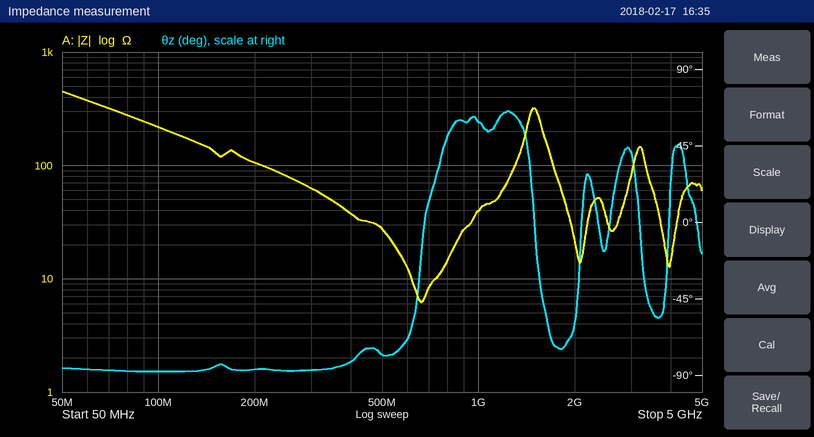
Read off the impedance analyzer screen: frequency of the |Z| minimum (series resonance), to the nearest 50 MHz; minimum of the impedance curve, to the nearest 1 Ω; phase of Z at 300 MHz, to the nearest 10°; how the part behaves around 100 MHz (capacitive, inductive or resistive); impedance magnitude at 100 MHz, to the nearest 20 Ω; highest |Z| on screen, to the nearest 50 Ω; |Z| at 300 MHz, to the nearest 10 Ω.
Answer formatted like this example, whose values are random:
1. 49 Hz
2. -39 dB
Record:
1. 650 MHz
2. 6 Ω
3. -90°
4. capacitive
5. 220 Ω
6. 450 Ω
7. 60 Ω
